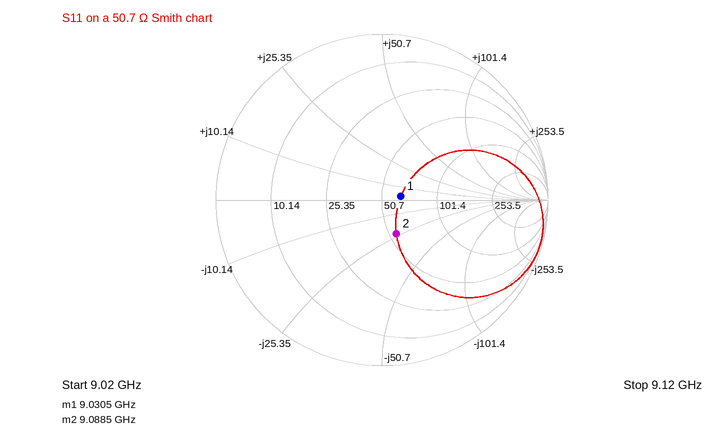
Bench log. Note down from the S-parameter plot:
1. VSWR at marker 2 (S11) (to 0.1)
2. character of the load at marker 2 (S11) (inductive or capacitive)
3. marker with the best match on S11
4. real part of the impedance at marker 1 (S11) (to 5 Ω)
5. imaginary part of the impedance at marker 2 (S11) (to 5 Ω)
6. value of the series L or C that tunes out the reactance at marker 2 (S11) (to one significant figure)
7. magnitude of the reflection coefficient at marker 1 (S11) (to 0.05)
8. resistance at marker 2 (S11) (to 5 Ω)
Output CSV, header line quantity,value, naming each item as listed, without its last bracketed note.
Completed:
quantity,value
VSWR at marker 2 (S11),1.6
character of the load at marker 2 (S11),capacitive
marker with the best match on S11,marker 1
real part of the impedance at marker 1 (S11),65 Ω
imaginary part of the impedance at marker 2 (S11),-25 Ω
value of the series L or C that tunes out the reactance at marker 2 (S11),400 pH
magnitude of the reflection coefficient at marker 1 (S11),0.10
resistance at marker 2 (S11),55 Ω
